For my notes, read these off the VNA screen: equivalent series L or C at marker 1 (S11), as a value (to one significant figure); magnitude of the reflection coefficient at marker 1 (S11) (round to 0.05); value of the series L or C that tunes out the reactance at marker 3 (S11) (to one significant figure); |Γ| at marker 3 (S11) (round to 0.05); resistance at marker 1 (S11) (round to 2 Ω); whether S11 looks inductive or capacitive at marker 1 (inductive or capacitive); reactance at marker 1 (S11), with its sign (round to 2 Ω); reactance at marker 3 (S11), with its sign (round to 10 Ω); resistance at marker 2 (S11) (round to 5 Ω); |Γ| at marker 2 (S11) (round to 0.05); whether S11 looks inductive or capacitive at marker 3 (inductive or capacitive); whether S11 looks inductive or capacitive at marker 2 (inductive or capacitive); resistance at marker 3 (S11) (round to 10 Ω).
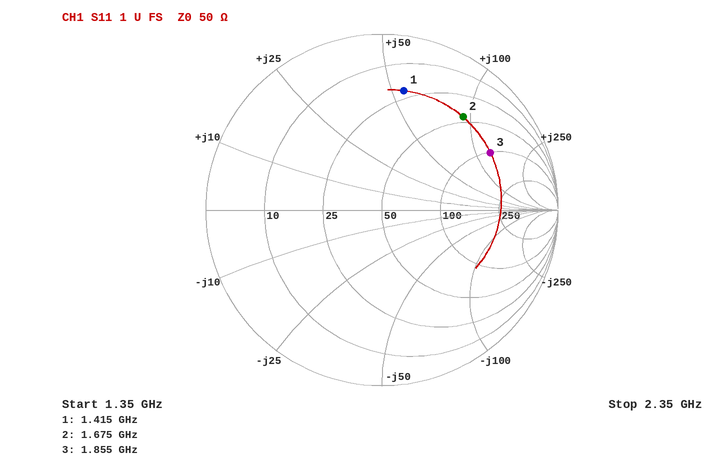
6 nH
0.70
700 fF
0.70
22 Ω
inductive
+56 Ω
+130 Ω
45 Ω
0.70
inductive
inductive
100 Ω
